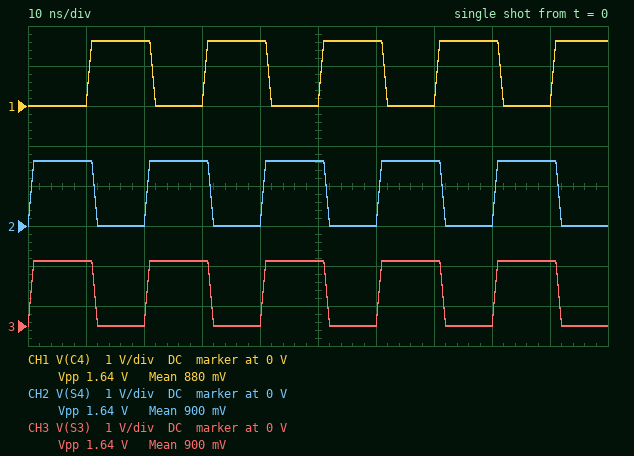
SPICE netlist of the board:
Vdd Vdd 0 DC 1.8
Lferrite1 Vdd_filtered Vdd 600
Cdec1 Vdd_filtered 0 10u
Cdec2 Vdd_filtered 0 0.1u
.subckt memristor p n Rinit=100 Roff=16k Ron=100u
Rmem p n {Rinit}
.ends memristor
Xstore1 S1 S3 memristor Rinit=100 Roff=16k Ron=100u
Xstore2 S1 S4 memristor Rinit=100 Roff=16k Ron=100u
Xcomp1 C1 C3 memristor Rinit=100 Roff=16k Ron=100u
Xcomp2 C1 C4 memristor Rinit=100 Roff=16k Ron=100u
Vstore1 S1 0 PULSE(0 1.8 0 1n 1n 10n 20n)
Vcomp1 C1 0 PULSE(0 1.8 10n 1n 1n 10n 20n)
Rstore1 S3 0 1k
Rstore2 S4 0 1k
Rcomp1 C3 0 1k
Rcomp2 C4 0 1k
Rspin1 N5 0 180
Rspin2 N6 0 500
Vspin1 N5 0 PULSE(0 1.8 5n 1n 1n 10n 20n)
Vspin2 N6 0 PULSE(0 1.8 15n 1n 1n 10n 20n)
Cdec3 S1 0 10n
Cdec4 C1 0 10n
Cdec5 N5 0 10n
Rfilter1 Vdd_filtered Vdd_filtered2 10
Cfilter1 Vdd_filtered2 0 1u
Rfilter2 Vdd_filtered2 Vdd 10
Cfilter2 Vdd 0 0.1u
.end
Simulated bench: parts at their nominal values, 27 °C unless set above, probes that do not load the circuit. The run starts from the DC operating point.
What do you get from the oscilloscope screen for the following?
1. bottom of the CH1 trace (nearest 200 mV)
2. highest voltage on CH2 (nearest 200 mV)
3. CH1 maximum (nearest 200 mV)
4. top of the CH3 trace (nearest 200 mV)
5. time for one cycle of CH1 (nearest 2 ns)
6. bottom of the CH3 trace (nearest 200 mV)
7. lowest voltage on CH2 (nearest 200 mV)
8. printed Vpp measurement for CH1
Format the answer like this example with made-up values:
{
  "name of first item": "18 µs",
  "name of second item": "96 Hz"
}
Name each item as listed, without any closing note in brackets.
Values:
{
  "bottom of the CH1 trace": "0 V",
  "highest voltage on CH2": "1.6 V",
  "CH1 maximum": "1.6 V",
  "top of the CH3 trace": "1.6 V",
  "time for one cycle of CH1": "20 ns",
  "bottom of the CH3 trace": "0 V",
  "lowest voltage on CH2": "0 V",
  "printed Vpp measurement for CH1": "1.64 V"
}
